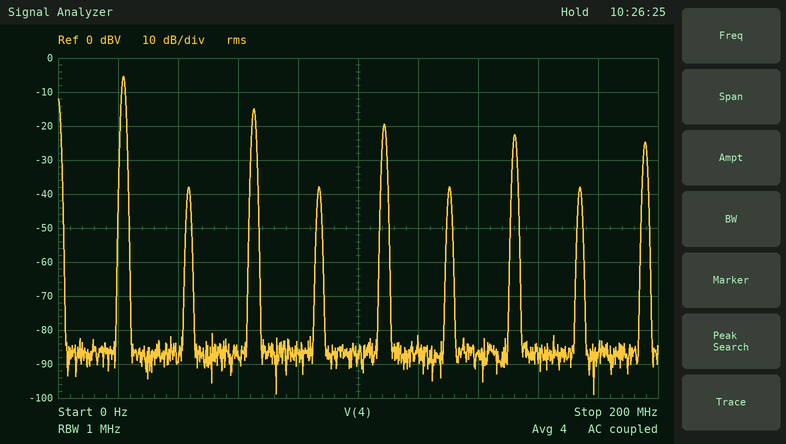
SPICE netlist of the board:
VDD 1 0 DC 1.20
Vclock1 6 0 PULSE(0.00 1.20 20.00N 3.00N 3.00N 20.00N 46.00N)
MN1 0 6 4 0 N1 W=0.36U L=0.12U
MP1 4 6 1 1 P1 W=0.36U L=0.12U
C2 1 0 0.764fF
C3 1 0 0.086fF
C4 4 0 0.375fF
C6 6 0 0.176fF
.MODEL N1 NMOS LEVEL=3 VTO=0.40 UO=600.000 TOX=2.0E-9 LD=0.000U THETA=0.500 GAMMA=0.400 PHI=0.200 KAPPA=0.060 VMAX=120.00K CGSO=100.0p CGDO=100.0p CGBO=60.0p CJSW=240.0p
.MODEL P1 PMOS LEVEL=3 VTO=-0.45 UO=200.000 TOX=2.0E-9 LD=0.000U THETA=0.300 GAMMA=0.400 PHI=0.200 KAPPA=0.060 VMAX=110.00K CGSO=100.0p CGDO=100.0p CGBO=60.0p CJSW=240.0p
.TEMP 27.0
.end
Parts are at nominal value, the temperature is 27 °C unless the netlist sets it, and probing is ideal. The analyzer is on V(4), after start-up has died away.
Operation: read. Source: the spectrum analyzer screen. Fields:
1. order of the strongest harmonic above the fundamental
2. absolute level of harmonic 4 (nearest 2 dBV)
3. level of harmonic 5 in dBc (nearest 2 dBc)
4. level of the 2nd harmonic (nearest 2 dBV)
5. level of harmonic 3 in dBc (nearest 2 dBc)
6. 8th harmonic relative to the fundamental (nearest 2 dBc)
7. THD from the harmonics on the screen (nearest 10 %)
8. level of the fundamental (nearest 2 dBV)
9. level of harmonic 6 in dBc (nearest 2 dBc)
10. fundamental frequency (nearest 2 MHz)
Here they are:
3
-38 dBV
-14 dBc
-38 dBV
-10 dBc
-32 dBc
40 %
-6 dBV
-32 dBc
22 MHz
